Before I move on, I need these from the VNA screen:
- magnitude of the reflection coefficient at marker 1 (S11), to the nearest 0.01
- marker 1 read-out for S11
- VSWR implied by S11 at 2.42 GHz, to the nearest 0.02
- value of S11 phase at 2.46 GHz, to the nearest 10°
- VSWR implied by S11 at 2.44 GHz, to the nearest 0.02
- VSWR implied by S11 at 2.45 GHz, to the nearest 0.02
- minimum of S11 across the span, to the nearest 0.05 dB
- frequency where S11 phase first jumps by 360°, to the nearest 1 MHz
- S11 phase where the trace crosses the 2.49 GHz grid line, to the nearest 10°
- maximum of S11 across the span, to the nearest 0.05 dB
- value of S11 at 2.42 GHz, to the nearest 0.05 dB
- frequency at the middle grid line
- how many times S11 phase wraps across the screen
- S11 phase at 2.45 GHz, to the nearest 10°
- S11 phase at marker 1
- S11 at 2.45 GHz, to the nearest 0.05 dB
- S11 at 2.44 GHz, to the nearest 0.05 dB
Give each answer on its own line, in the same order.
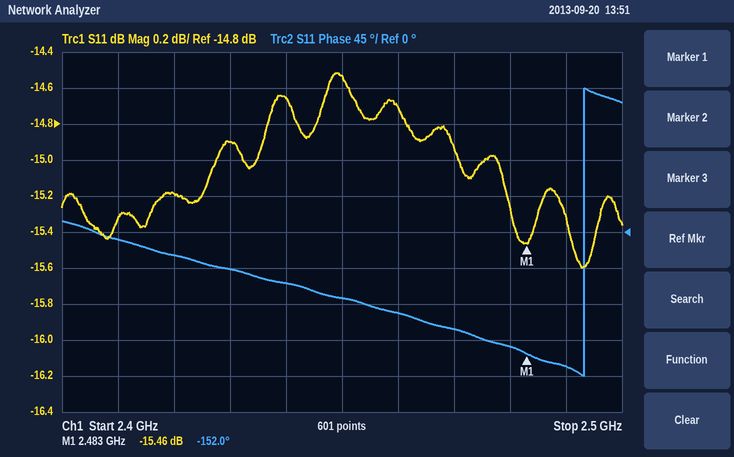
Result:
0.17
-15.46 dB
1.42
-100°
1.46
1.46
-15.60 dB
2.493 GHz
-170°
-14.50 dB
-15.20 dB
2.45 GHz
1
-80°
-152.0°
-14.55 dB
-14.65 dB
